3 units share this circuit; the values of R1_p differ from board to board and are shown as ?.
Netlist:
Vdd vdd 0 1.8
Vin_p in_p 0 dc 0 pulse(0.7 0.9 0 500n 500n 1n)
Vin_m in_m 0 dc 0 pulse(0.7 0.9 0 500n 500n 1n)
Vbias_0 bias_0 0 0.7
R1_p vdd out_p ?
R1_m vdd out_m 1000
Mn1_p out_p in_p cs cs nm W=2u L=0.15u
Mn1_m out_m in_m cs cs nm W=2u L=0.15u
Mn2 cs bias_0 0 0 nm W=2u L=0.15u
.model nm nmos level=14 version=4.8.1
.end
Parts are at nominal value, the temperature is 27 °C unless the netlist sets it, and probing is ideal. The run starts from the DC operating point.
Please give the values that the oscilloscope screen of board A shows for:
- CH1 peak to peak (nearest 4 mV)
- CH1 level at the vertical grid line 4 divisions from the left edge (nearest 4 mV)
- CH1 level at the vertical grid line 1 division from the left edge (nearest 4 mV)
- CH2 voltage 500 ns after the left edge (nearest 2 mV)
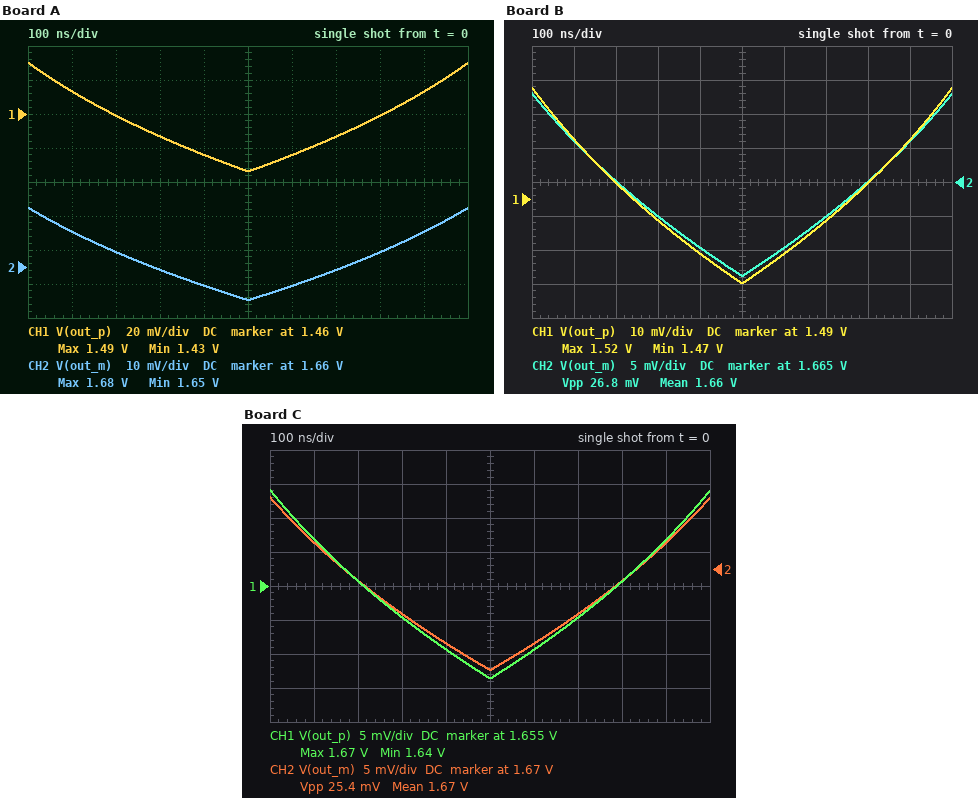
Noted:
64 mV
1.436 V
1.472 V
1.650 V
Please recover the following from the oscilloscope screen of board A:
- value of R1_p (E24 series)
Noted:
2.7 kΩ
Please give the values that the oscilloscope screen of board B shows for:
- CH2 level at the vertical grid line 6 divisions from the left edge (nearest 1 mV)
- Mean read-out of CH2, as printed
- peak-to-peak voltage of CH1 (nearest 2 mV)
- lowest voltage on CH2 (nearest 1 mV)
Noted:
1.655 V
1.66 V
58 mV
1.651 V
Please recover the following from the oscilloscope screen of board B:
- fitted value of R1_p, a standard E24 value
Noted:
2.4 kΩ
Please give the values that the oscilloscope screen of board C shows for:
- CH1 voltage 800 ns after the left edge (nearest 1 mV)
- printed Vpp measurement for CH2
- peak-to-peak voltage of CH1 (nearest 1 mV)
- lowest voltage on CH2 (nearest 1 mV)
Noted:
1.656 V
25.4 mV
28 mV
1.655 V
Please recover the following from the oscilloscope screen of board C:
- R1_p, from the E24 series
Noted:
1.1 kΩ
